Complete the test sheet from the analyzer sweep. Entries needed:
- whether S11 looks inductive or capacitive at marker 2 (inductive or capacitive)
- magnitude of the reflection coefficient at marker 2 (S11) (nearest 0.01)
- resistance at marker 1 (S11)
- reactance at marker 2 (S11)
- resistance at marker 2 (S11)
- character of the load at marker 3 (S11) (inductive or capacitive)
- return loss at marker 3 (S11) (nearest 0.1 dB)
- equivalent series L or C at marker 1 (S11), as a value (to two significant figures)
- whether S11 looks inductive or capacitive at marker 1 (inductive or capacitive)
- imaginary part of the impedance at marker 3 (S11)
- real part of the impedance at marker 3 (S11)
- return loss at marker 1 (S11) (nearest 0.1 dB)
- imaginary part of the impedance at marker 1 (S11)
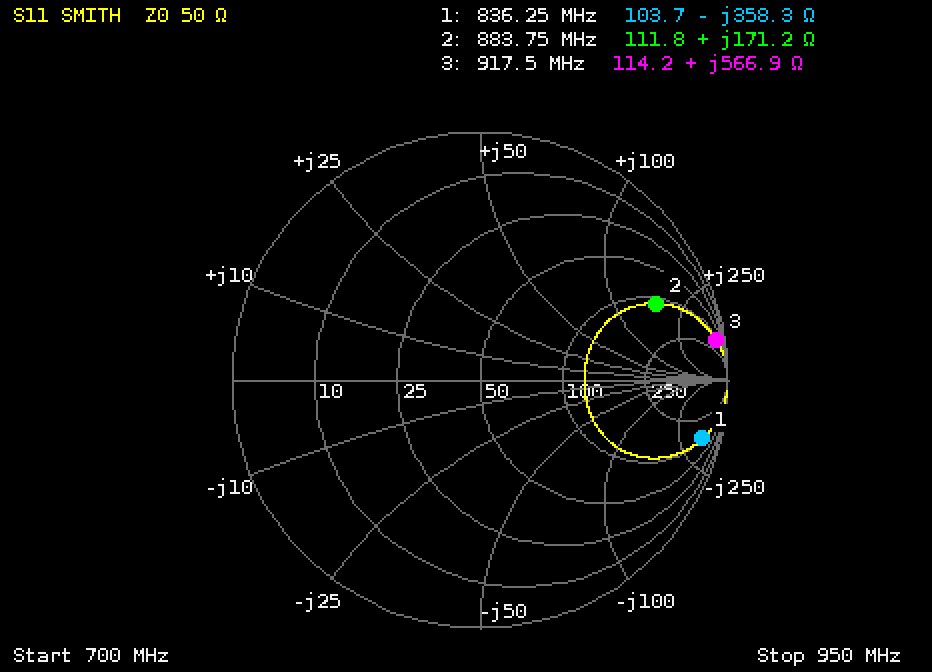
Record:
inductive
0.77
103.7 Ω
+171.2 Ω
111.8 Ω
inductive
0.3 dB
530 fF
capacitive
+566.9 Ω
114.2 Ω
0.6 dB
-358.3 Ω
